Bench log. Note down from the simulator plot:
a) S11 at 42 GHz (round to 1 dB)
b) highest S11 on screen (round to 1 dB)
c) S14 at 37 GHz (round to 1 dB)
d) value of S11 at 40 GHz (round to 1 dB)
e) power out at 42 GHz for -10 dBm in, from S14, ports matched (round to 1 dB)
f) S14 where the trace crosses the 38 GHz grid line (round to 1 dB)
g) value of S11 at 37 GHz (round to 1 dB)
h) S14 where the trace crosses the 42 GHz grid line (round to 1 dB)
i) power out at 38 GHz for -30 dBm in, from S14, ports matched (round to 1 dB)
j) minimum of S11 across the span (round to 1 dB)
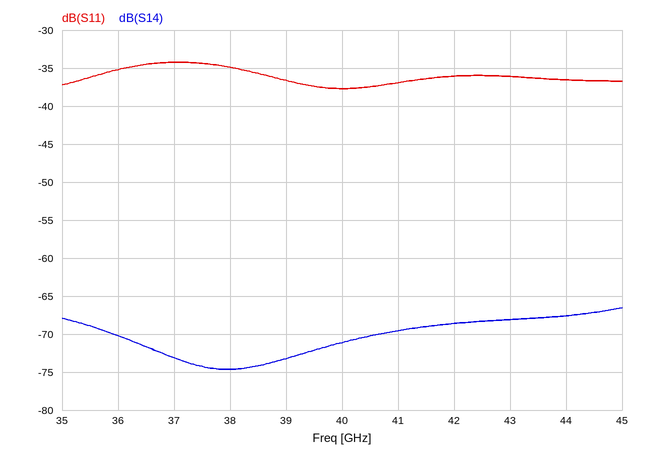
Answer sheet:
-36 dB
-34 dB
-73 dB
-38 dB
-79 dBm
-75 dB
-34 dB
-69 dB
-105 dBm
-38 dB
